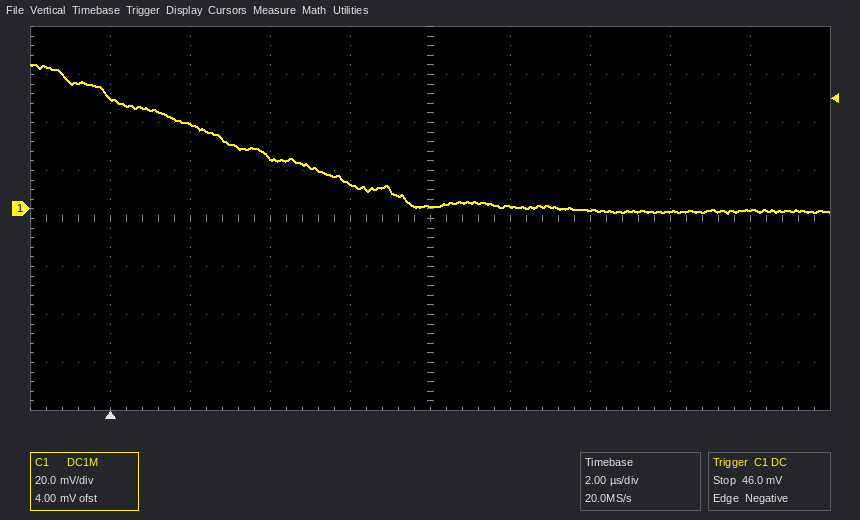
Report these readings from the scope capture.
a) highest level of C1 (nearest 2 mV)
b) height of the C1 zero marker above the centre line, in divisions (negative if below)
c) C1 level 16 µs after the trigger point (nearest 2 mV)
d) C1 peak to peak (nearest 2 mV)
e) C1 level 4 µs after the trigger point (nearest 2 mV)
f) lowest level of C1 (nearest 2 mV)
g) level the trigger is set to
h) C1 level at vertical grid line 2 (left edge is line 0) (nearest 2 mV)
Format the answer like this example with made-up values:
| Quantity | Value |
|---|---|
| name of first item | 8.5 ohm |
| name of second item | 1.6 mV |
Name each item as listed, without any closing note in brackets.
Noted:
| Quantity | Value |
|---|---|
| highest level of C1 | 60 mV |
| height of the C1 zero marker above the centre line, in divisions | +0.2 div |
| C1 level 16 µs after the trigger point | 0 mV |
| C1 peak to peak | 62 mV |
| C1 level 4 µs after the trigger point | 22 mV |
| lowest level of C1 | -2 mV |
| level the trigger is set to | 46.0 mV |
| C1 level at vertical grid line 2 (left edge is line 0) | 36 mV |
